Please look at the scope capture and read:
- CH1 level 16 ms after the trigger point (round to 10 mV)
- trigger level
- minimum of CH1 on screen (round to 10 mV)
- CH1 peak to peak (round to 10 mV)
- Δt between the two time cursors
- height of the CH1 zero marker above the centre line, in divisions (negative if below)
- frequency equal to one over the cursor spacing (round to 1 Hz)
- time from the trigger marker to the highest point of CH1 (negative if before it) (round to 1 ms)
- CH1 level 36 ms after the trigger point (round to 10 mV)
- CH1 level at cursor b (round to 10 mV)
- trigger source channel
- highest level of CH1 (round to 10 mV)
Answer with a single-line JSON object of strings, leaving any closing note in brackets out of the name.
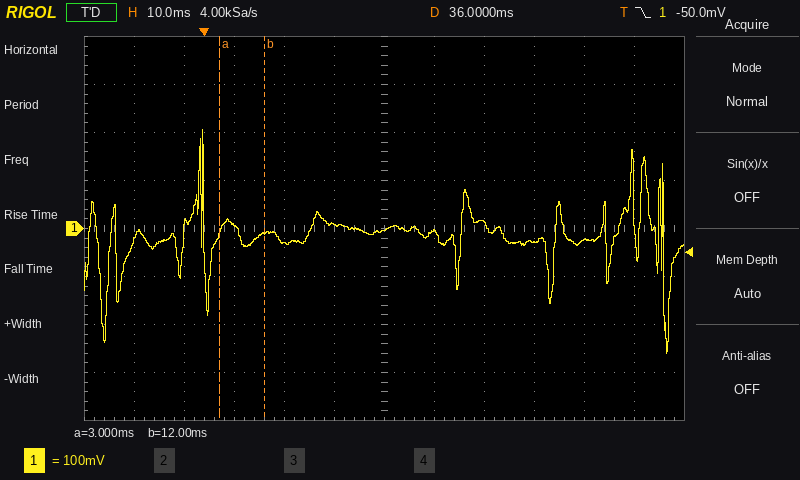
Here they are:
{"CH1 level 16 ms after the trigger point": "-30 mV", "trigger level": "-50.0 mV", "minimum of CH1 on screen": "-260 mV", "CH1 peak to peak": "470 mV", "Δt between the two time cursors": "9 ms", "height of the CH1 zero marker above the centre line, in divisions": "0.0 div", "frequency equal to one over the cursor spacing": "111 Hz", "time from the trigger marker to the highest point of CH1 (negative if before it)": "0 ms", "CH1 level 36 ms after the trigger point": "0 mV", "CH1 level at cursor b": "-10 mV", "trigger source channel": "CH1", "highest level of CH1": "210 mV"}
